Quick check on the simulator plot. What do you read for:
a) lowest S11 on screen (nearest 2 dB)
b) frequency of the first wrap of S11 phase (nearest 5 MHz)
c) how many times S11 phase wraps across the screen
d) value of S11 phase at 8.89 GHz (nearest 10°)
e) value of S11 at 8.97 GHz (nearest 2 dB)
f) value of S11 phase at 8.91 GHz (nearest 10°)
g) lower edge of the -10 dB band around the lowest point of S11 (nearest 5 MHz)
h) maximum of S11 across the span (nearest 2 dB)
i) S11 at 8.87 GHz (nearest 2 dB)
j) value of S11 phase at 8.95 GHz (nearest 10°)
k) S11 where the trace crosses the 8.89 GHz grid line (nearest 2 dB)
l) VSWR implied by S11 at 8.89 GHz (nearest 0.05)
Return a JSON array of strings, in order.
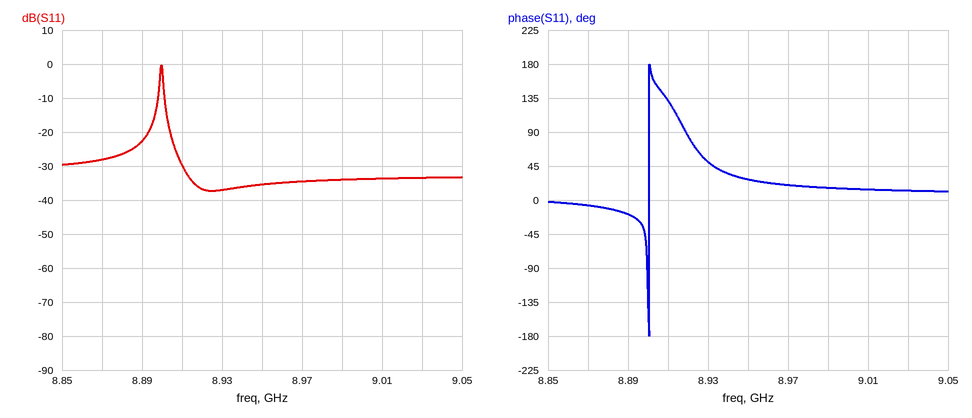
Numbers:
["-38 dB", "8.900 GHz", "1", "-20°", "-34 dB", "130°", "8.900 GHz", "0 dB", "-28 dB", "30°", "-22 dB", "1.15"]
